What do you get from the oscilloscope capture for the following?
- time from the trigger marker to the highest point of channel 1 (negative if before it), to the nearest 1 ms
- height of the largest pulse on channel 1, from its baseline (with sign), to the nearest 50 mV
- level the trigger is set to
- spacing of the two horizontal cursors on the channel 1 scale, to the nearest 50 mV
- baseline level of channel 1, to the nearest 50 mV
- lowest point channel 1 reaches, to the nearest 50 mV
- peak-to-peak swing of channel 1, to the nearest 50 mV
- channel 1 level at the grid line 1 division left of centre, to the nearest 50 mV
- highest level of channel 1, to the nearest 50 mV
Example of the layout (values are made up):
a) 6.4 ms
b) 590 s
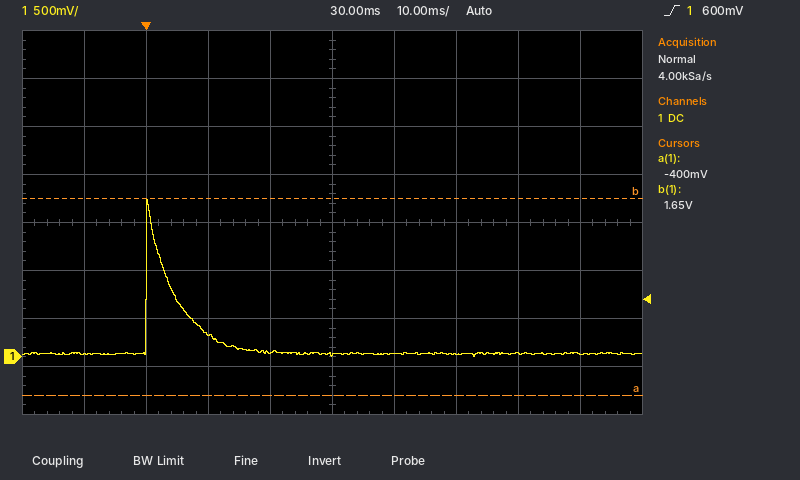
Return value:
a) 0 ms
b) +1.60 V
c) 600 mV
d) 2.05 V
e) 50 mV
f) 0 mV
g) 1.65 V
h) 50 mV
i) 1.65 V
